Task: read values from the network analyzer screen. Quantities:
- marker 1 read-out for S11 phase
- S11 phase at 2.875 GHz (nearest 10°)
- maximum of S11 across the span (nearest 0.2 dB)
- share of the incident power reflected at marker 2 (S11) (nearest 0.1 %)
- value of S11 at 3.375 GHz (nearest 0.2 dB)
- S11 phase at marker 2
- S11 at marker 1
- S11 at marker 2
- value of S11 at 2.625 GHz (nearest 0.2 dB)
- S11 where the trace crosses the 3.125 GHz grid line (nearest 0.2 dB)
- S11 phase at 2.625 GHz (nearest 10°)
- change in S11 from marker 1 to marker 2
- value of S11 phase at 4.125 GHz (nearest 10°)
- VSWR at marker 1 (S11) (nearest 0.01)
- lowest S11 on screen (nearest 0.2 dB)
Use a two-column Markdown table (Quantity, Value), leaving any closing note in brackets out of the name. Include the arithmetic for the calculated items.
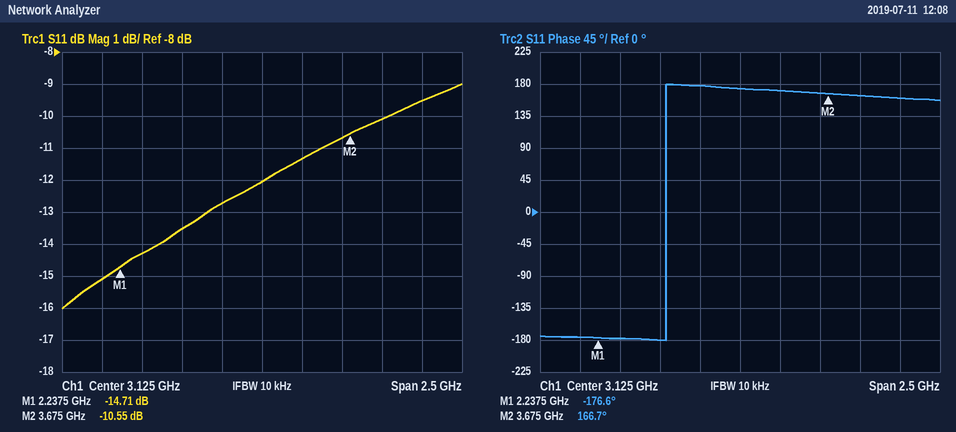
| Quantity | Value |
|---|---|
| marker 1 read-out for S11 phase | -176.6° |
| S11 phase at 2.875 GHz | 180° |
| maximum of S11 across the span | -9.0 dB |
| share of the incident power reflected at marker 2 (S11) | 10^(-10.55/10) ≈ 8.8 % |
| value of S11 at 3.375 GHz | -11.4 dB |
| S11 phase at marker 2 | 166.7° |
| S11 at marker 1 | -14.71 dB |
| S11 at marker 2 | -10.55 dB |
| value of S11 at 2.625 GHz | -13.6 dB |
| S11 where the trace crosses the 3.125 GHz grid line | -12.0 dB |
| S11 phase at 2.625 GHz | -180° |
| change in S11 from marker 1 to marker 2 | -10.55 − (-14.71) = 4.16 dB |
| value of S11 phase at 4.125 GHz | 160° |
| VSWR at marker 1 (S11) | (1 + 0.1839)/(1 − 0.1839) ≈ 1.45 |
| lowest S11 on screen | -16.0 dB |
